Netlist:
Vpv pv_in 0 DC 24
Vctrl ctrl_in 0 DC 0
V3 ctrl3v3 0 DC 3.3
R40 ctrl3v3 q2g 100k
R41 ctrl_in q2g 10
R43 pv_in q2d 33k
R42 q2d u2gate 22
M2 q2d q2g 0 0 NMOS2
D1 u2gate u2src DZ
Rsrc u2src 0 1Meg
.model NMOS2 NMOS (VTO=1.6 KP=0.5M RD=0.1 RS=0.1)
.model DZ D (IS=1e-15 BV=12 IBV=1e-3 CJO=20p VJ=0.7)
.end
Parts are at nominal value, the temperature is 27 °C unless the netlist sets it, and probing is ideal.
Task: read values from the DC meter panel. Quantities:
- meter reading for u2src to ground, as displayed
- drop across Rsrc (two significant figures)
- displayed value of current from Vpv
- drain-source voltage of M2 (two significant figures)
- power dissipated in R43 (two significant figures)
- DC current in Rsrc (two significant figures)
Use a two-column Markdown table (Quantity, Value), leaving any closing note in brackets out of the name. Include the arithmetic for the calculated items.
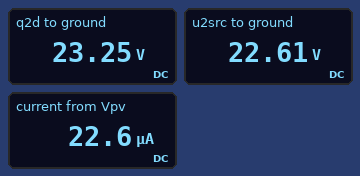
| Quantity | Value |
|---|---|
| meter reading for u2src to ground, as displayed | 22.61 V |
| drop across Rsrc | 22.61 V = 23 V |
| displayed value of current from Vpv | 22.6 µA |
| drain-source voltage of M2 | 23.25 V = 23 V |
| power dissipated in R43 | (24 V - 23.25 V)^2 / 33 kΩ = 17 µW |
| DC current in Rsrc | (22.61 V) / 1 MΩ = 23 µA |
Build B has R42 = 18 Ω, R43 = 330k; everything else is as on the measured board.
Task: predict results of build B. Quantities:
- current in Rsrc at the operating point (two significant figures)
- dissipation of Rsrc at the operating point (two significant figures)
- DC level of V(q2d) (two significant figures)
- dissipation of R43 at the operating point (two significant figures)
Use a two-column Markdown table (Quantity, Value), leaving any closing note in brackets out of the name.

| Quantity | Value |
|---|---|
| current in Rsrc at the operating point | 18 µA |
| dissipation of Rsrc at the operating point | 310 µW |
| DC level of V(q2d) | 18 V |
| dissipation of R43 at the operating point | 100 µW |
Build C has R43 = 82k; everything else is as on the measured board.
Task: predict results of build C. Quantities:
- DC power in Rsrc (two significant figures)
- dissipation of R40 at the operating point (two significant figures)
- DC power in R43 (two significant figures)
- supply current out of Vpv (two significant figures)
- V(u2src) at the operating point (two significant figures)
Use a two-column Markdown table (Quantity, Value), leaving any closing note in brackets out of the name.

| Quantity | Value |
|---|---|
| DC power in Rsrc | 470 µW |
| dissipation of R40 at the operating point | 110 µW |
| DC power in R43 | 38 µW |
| supply current out of Vpv | 22 µA |
| V(u2src) at the operating point | 22 V |
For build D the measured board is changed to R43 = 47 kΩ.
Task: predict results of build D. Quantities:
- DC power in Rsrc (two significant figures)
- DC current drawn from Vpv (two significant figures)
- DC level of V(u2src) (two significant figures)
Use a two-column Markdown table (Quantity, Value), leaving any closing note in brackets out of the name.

| Quantity | Value |
|---|---|
| DC power in Rsrc | 500 µW |
| DC current drawn from Vpv | 22 µA |
| DC level of V(u2src) | 22 V |
